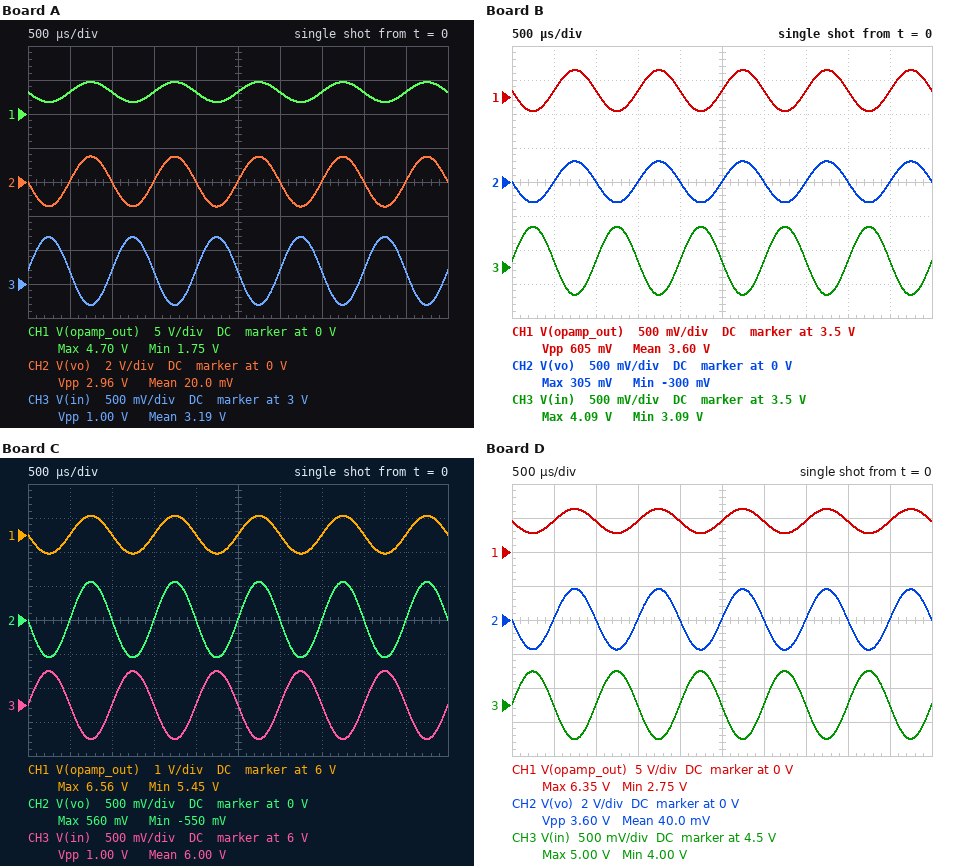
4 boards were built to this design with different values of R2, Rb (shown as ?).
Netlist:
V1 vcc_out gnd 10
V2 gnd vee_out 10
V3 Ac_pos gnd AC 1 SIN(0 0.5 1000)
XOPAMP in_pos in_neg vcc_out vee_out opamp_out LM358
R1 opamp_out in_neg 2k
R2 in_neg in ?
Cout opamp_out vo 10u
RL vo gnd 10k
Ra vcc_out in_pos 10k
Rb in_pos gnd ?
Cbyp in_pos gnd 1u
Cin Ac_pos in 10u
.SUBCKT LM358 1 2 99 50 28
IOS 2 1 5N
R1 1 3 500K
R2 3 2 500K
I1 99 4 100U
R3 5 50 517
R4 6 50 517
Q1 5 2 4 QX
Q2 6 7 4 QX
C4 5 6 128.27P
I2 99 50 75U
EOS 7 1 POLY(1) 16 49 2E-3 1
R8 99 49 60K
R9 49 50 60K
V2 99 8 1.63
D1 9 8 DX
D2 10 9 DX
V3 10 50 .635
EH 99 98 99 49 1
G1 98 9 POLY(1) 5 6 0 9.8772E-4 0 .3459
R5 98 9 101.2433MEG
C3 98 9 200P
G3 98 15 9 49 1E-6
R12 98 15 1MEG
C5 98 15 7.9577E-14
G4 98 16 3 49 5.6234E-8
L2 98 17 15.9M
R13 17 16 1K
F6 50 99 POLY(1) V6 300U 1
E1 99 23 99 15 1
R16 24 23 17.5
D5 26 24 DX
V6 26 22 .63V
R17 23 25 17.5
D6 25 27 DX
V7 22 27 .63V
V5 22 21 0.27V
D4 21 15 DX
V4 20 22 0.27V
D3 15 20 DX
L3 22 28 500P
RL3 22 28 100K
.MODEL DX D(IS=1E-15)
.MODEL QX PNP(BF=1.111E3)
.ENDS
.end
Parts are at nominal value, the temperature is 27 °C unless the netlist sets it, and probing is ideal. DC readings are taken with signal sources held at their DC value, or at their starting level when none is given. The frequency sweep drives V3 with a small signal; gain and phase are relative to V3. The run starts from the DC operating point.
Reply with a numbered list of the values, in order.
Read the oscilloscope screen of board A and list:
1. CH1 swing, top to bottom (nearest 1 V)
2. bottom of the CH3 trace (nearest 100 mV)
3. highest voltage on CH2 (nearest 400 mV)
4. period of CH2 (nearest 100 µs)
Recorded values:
1. 3 V
2. 2.7 V
3. 1.6 V
4. 1.0 ms
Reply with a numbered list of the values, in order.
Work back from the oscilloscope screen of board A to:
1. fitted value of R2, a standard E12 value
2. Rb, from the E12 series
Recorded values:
1. 680 Ω
2. 4.7 kΩ
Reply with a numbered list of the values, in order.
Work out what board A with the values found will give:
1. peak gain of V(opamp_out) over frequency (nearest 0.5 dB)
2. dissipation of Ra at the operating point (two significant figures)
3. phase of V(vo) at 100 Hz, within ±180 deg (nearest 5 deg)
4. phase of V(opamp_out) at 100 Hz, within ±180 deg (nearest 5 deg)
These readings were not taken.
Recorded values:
1. 9.5 dB
2. 4.6 mW
3. -165 deg
4. -165 deg
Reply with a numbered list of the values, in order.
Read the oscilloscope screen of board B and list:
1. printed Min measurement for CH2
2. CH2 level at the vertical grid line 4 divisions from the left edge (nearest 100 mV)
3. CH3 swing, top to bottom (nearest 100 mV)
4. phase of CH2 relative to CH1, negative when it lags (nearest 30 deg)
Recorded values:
1. -300 mV
2. 0 V
3. 1.0 V
4. 0 deg
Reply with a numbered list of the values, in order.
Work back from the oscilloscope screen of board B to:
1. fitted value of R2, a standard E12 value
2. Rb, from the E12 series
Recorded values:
1. 3.3 kΩ
2. 5.6 kΩ
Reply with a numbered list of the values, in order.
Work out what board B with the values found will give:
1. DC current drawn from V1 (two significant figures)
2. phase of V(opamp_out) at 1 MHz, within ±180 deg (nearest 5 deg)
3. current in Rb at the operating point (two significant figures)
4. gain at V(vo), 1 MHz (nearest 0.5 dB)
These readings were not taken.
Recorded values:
1. 720 µA
2. 25 deg
3. 640 µA
4. -9.5 dB
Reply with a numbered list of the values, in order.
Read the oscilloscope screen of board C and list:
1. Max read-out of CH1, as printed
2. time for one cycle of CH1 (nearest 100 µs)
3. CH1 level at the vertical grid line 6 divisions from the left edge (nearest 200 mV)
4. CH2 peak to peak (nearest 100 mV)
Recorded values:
1. 6.56 V
2. 1.0 ms
3. 6.0 V
4. 1.1 V
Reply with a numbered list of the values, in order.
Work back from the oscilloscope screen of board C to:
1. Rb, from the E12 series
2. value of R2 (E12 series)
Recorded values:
1. 15 kΩ
2. 1.8 kΩ
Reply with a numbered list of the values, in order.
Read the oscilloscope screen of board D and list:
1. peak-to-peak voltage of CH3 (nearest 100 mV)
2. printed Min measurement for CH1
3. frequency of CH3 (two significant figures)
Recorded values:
1. 1.0 V
2. 2.75 V
3. 1.0 kHz
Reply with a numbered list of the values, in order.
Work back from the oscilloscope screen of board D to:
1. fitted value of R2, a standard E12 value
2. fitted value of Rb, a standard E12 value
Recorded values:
1. 560 Ω
2. 8.2 kΩ
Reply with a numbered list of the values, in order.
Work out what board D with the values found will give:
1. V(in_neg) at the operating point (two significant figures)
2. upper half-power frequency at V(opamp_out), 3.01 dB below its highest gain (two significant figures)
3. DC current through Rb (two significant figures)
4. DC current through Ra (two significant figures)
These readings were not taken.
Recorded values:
1. 4.5 V
2. 190 kHz
3. 550 µA
4. 550 µA
